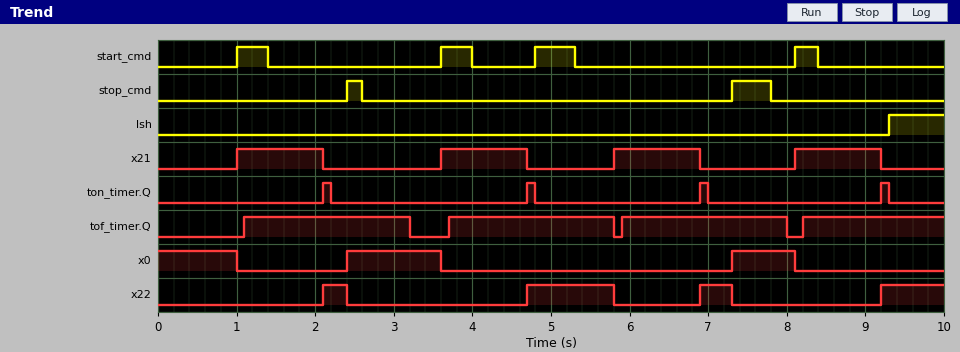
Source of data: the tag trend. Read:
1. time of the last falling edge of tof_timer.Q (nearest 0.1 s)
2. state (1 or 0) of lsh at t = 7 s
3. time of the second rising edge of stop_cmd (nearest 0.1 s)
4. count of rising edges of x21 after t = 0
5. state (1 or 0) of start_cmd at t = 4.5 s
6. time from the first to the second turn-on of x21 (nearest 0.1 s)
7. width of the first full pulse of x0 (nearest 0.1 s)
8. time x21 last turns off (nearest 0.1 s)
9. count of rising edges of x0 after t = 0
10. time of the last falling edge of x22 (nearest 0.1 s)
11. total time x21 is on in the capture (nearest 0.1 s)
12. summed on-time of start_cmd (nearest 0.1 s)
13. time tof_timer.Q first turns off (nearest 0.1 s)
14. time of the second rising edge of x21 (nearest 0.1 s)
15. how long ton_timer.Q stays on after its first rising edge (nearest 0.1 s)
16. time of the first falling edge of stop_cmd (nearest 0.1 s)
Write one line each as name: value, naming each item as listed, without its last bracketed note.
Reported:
time of the last falling edge of tof_timer.Q: 8.0 s
state (1 or 0) of lsh at t = 7 s: 0
time of the second rising edge of stop_cmd: 7.3 s
count of rising edges of x21 after t = 0: 4
state (1 or 0) of start_cmd at t = 4.5 s: 0
time from the first to the second turn-on of x21: 2.6 s
width of the first full pulse of x0: 1.2 s
time x21 last turns off: 9.2 s
count of rising edges of x0 after t = 0: 2
time of the last falling edge of x22: 7.3 s
total time x21 is on in the capture: 4.4 s
summed on-time of start_cmd: 1.6 s
time tof_timer.Q first turns off: 3.2 s
time of the second rising edge of x21: 3.6 s
how long ton_timer.Q stays on after its first rising edge: 0.1 s
time of the first falling edge of stop_cmd: 2.6 s
